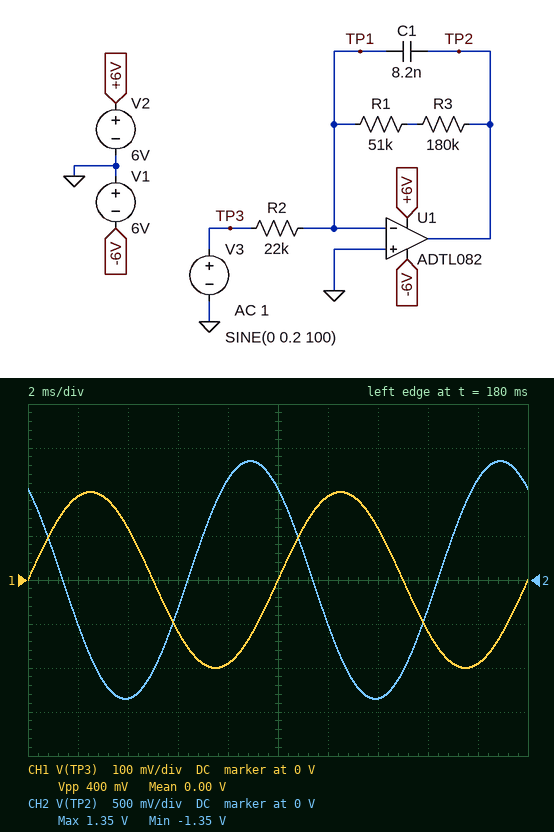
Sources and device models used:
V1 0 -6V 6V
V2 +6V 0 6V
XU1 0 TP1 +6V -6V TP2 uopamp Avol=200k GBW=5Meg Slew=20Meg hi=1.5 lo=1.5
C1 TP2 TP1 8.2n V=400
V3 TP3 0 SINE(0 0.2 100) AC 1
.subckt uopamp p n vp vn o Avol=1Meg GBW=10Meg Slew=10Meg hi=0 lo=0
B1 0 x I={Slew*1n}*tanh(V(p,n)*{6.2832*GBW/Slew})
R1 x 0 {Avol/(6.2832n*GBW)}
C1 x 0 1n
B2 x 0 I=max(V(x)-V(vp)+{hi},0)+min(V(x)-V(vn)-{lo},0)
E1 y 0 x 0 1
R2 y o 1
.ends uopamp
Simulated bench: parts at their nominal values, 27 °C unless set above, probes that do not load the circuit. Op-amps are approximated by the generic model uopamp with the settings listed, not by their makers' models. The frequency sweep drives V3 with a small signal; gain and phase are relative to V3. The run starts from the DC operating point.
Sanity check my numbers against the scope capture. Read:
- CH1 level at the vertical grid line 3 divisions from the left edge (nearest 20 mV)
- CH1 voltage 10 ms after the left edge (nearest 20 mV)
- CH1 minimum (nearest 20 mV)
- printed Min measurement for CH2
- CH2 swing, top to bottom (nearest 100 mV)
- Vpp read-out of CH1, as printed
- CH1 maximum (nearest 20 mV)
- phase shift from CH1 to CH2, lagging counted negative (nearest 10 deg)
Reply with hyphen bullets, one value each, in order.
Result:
- -120 mV
- 0 V
- -200 mV
- -1.35 V
- 2.7 V
- 400 mV
- 200 mV
- 130 deg
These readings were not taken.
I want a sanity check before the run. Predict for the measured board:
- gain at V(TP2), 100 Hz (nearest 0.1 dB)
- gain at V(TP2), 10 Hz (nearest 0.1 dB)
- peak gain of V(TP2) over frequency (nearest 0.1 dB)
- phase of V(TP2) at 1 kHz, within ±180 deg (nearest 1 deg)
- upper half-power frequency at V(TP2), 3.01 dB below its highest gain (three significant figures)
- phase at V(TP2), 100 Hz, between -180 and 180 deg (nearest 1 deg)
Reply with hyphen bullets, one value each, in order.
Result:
- 16.6 dB
- 20.4 dB
- 20.4 dB
- 95 deg
- 84.0 Hz
- 130 deg
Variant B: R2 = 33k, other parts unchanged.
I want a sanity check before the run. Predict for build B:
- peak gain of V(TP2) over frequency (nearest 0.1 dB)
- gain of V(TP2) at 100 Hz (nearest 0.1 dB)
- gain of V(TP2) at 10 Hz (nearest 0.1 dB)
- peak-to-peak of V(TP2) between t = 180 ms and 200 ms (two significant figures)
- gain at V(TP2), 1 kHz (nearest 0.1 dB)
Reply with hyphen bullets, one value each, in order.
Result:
- 16.9 dB
- 13.1 dB
- 16.8 dB
- 1.8 V
- -4.6 dB
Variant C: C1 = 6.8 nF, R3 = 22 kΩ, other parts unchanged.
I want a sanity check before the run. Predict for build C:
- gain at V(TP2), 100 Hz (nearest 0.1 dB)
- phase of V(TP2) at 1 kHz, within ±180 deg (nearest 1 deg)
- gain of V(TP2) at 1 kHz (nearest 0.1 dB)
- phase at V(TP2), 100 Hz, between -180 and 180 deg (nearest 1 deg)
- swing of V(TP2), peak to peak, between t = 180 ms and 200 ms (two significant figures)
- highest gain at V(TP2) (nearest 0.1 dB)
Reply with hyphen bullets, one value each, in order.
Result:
- 10.0 dB
- 108 deg
- 0.1 dB
- 163 deg
- 1.3 V
- 10.4 dB
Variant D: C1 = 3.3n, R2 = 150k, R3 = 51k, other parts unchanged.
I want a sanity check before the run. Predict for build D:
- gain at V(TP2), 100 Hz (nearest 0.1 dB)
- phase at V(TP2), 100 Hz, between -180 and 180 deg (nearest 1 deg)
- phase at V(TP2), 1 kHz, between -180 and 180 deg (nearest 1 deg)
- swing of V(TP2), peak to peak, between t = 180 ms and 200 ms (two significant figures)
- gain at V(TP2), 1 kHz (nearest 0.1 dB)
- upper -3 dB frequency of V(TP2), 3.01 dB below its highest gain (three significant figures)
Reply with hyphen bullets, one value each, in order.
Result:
- -3.5 dB
- 168 deg
- 115 deg
- 270 mV
- -10.7 dB
- 473 Hz
